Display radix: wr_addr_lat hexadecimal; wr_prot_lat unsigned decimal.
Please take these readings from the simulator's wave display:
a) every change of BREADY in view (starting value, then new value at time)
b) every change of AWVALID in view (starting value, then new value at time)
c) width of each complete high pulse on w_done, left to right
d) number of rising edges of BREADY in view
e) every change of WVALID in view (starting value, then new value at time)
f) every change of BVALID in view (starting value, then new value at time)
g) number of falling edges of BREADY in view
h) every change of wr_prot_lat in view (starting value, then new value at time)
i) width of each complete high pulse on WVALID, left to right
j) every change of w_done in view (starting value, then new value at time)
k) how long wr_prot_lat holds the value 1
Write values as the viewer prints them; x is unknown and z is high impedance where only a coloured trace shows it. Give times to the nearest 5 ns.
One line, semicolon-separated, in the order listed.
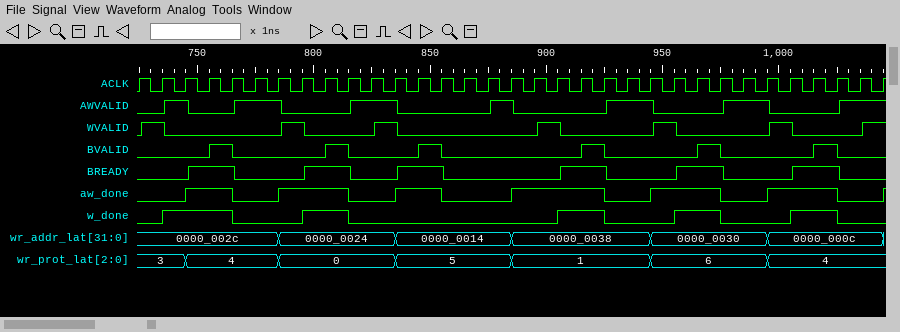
0, 1 at 745 ns, 0 at 765 ns, 1 at 795 ns, 0 at 815 ns, 1 at 835 ns, 0 at 855 ns, 1 at 905 ns, 0 at 925 ns, 1 at 955 ns, 0 at 975 ns, 1 at 1005 ns, 0 at 1025 ns; 0, 1 at 735 ns, 0 at 745 ns, 1 at 765 ns, 0 at 785 ns, 1 at 815 ns, 0 at 835 ns, 1 at 875 ns, 0 at 885 ns, 1 at 925 ns, 0 at 945 ns, 1 at 975 ns, 0 at 995 ns, 1 at 1025 ns; 30 ns, 20 ns, 20 ns, 20 ns, 20 ns; 6; 0, 1 at 725 ns, 0 at 735 ns, 1 at 785 ns, 0 at 795 ns, 1 at 825 ns, 0 at 835 ns, 1 at 895 ns, 0 at 905 ns, 1 at 945 ns, 0 at 955 ns, 1 at 995 ns, 0 at 1005 ns, 1 at 1035 ns; 0, 1 at 755 ns, 0 at 765 ns, 1 at 805 ns, 0 at 815 ns, 1 at 845 ns, 0 at 855 ns, 1 at 915 ns, 0 at 925 ns, 1 at 965 ns, 0 at 975 ns, 1 at 1015 ns, 0 at 1025 ns; 6; 3, 4 at 745 ns, 0 at 785 ns, 5 at 835 ns, 1 at 885 ns, 6 at 945 ns, 4 at 995 ns; 10 ns, 10 ns, 10 ns, 10 ns, 10 ns, 10 ns; 0, 1 at 735 ns, 0 at 765 ns, 1 at 795 ns, 0 at 815 ns, 1 at 905 ns, 0 at 925 ns, 1 at 955 ns, 0 at 975 ns, 1 at 1005 ns, 0 at 1025 ns; 60 ns
